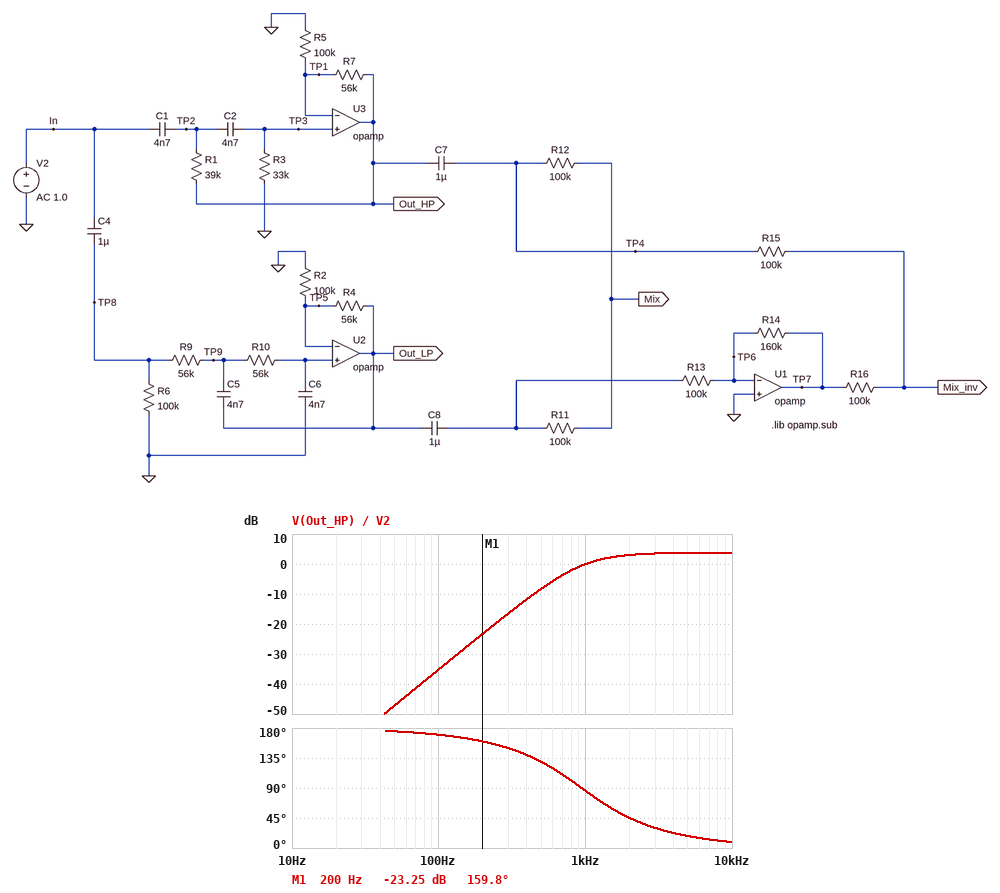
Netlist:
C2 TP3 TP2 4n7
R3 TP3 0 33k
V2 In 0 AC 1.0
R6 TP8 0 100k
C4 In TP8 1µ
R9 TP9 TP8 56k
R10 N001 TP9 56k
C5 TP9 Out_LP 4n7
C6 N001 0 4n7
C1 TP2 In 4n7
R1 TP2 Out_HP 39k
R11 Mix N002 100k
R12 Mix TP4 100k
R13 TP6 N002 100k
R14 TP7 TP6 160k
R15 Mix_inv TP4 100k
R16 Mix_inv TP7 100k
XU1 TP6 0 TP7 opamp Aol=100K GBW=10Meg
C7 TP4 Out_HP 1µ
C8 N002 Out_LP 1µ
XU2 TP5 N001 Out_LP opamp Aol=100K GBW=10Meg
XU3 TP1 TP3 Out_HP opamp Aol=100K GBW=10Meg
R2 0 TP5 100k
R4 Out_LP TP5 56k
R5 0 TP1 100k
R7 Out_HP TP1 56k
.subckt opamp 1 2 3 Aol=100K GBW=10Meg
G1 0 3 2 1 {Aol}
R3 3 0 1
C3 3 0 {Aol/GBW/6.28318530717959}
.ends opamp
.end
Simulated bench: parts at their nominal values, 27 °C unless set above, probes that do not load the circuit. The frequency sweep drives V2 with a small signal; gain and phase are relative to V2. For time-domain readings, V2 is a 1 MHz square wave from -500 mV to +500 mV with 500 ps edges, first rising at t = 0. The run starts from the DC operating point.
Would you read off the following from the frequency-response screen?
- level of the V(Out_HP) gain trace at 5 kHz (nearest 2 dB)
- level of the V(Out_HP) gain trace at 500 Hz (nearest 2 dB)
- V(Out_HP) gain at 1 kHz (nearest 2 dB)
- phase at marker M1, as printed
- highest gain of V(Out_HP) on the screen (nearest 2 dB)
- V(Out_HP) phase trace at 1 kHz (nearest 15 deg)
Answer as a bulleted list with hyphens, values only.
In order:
- 4 dB
- -8 dB
- 0 dB
- 159.8 deg
- 4 dB
- 90 deg
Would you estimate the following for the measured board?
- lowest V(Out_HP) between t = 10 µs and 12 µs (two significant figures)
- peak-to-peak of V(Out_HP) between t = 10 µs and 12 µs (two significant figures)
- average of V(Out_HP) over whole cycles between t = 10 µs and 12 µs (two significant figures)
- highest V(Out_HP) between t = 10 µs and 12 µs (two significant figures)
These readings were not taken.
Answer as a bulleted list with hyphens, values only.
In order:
- -89 mV
- 1.6 V
- 700 mV
- 1.5 V
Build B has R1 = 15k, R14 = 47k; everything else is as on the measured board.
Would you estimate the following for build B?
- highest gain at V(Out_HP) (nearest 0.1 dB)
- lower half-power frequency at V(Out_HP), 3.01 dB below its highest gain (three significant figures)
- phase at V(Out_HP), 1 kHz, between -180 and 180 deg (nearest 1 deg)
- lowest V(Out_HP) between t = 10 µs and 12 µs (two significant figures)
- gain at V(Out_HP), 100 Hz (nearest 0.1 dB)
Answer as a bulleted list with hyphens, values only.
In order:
- 9.9 dB
- 1.30 kHz
- 149 deg
- -50 mV
- -43.4 dB
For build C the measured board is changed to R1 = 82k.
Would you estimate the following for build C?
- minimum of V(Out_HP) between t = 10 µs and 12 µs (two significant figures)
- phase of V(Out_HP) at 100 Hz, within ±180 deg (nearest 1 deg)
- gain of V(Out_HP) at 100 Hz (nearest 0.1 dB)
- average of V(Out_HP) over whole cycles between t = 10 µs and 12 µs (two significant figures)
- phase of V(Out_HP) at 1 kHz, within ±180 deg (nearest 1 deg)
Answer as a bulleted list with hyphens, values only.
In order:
- -100 mV
- 156 deg
- -29.2 dB
- 690 mV
- 72 deg
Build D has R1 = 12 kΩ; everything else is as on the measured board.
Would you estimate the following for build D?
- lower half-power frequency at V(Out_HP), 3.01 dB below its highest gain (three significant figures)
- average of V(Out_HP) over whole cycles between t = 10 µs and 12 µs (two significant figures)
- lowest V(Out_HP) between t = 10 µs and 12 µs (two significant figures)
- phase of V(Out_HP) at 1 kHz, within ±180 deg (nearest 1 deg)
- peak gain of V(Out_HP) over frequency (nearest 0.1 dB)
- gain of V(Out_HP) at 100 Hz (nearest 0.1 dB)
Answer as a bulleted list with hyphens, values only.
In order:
- 1.53 kHz
- 750 mV
- -34 mV
- 166 deg
- 15.1 dB
- -45.3 dB
